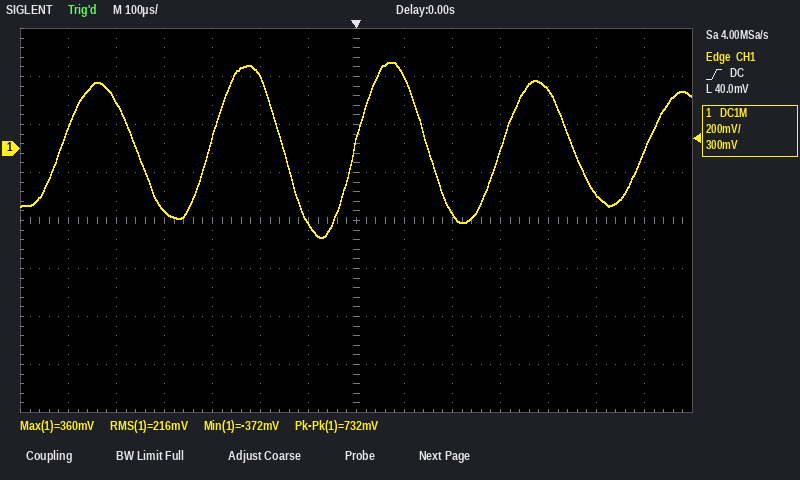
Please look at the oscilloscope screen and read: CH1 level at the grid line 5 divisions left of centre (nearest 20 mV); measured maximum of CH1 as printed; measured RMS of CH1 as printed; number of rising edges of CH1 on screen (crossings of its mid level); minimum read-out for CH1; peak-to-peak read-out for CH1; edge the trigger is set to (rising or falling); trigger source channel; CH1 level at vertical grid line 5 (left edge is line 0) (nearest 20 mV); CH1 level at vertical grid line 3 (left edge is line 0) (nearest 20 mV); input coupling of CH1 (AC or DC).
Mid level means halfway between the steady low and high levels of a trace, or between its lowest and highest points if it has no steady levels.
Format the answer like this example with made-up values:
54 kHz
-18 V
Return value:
200 mV
360 mV
216 mV
5
-372 mV
732 mV
rising
CH1
300 mV
-260 mV
DC
